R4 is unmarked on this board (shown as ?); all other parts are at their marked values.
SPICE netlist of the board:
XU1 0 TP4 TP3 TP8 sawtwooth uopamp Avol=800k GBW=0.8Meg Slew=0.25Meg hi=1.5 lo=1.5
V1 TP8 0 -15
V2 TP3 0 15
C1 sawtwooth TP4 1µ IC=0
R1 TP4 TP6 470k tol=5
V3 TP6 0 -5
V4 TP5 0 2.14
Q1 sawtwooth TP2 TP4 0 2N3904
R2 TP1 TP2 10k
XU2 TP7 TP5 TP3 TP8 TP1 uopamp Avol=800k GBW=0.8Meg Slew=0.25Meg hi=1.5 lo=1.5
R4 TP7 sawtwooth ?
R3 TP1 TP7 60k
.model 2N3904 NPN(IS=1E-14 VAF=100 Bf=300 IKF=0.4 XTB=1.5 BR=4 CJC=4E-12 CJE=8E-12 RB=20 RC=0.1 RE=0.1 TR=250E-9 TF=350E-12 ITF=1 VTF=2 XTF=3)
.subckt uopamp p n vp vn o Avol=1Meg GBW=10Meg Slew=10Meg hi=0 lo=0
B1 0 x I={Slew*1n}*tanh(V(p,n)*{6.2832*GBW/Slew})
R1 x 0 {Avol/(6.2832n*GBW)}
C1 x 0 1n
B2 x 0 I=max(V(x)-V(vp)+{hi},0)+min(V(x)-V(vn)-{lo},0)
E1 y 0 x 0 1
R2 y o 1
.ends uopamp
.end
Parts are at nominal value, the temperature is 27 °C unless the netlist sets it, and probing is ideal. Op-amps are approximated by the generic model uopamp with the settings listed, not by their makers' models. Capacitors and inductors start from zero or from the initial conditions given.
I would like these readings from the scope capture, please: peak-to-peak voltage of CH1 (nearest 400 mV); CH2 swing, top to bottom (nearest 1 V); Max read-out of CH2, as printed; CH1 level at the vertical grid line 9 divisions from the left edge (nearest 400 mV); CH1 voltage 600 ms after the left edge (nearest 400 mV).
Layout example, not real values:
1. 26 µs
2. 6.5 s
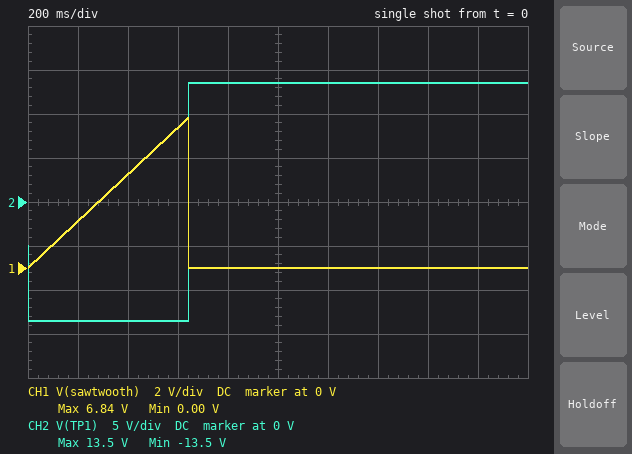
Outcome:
1. 6.8 V
2. 27 V
3. 13.5 V
4. 0 V
5. 6.4 V
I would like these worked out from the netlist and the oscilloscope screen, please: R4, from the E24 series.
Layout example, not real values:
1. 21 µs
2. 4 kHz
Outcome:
1. 18 kΩ
